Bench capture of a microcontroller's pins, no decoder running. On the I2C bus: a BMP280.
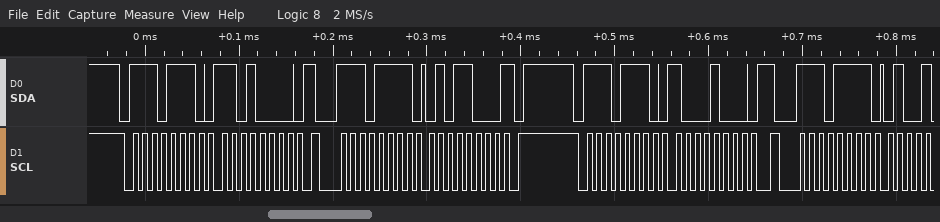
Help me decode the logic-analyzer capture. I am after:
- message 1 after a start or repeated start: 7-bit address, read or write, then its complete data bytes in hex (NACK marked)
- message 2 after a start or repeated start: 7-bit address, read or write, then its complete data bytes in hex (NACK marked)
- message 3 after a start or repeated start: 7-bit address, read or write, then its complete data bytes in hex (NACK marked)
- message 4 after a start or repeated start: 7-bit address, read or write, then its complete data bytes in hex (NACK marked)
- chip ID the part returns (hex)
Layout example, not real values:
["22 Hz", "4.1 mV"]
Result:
["0x77 write: D0", "0x77 read: 58 NACK", "0x77 write: 88", "0x77 read", "0x58"]
